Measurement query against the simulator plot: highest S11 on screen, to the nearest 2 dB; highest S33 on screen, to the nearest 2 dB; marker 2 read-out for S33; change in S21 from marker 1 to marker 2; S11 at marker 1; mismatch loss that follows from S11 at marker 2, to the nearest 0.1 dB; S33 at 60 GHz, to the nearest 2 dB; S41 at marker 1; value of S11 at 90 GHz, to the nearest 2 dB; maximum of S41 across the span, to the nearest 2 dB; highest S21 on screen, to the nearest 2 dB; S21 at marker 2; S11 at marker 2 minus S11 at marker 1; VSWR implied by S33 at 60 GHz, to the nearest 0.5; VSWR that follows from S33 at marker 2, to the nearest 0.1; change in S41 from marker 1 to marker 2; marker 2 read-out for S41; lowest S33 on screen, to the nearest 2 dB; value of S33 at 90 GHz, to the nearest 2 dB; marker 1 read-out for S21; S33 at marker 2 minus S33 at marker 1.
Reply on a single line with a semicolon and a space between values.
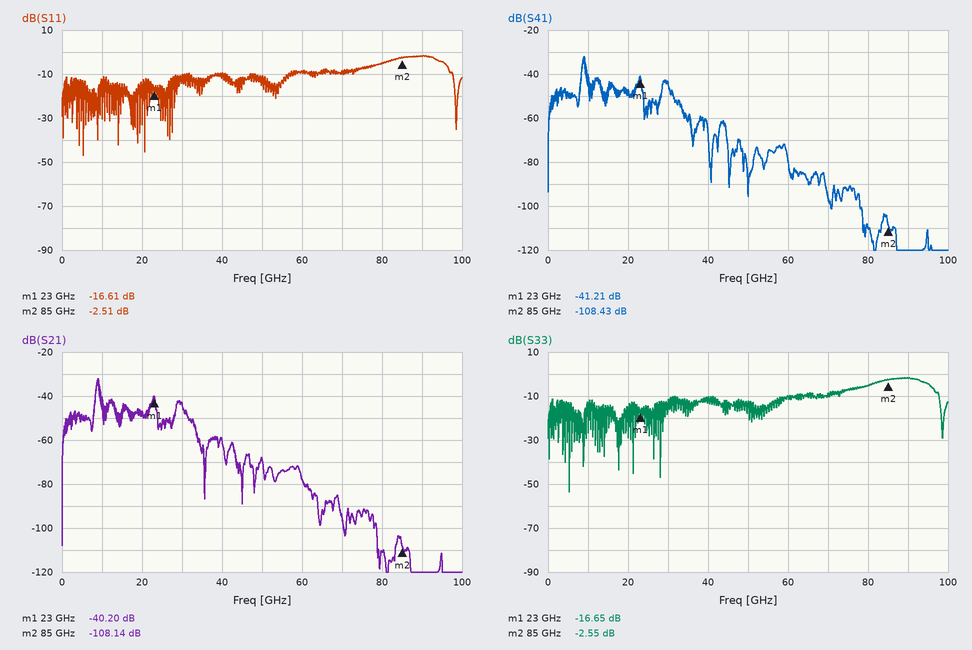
-2 dB; -2 dB; -2.55 dB; -67.94 dB; -16.61 dB; 3.6 dB; -10 dB; -41.21 dB; -2 dB; -32 dB; -32 dB; -108.14 dB; 14.10 dB; 2.0; 6.9; -67.22 dB; -108.43 dB; -54 dB; -2 dB; -40.20 dB; 14.10 dB
